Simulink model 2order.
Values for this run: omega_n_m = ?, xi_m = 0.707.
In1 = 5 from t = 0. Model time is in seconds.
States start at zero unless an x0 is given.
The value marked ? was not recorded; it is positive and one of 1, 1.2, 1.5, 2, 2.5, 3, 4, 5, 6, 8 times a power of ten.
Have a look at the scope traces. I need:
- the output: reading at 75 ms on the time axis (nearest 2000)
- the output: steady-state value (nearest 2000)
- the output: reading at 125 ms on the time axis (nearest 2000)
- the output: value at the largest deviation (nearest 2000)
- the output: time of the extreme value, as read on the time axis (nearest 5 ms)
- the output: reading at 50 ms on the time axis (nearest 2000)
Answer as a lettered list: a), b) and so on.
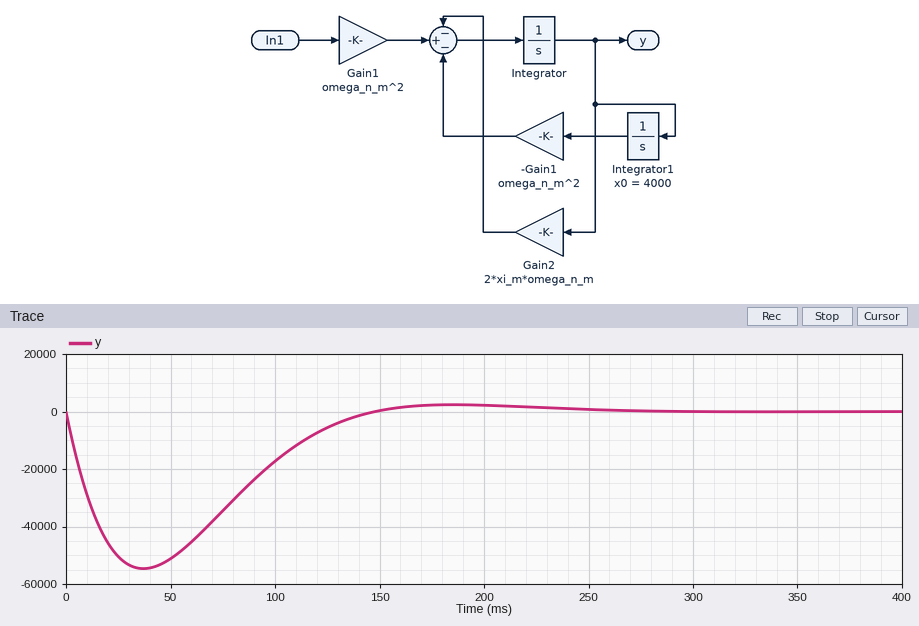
a) -34000
b) 0
c) -6000
d) -54000
e) 35 ms
f) -52000
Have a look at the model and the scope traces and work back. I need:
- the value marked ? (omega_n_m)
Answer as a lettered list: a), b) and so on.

a) 30
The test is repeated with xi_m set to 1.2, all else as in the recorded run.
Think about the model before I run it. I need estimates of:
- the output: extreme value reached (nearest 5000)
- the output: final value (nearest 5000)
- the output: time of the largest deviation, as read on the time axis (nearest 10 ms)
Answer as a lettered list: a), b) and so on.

a) -40000
b) 0
c) 30 ms
